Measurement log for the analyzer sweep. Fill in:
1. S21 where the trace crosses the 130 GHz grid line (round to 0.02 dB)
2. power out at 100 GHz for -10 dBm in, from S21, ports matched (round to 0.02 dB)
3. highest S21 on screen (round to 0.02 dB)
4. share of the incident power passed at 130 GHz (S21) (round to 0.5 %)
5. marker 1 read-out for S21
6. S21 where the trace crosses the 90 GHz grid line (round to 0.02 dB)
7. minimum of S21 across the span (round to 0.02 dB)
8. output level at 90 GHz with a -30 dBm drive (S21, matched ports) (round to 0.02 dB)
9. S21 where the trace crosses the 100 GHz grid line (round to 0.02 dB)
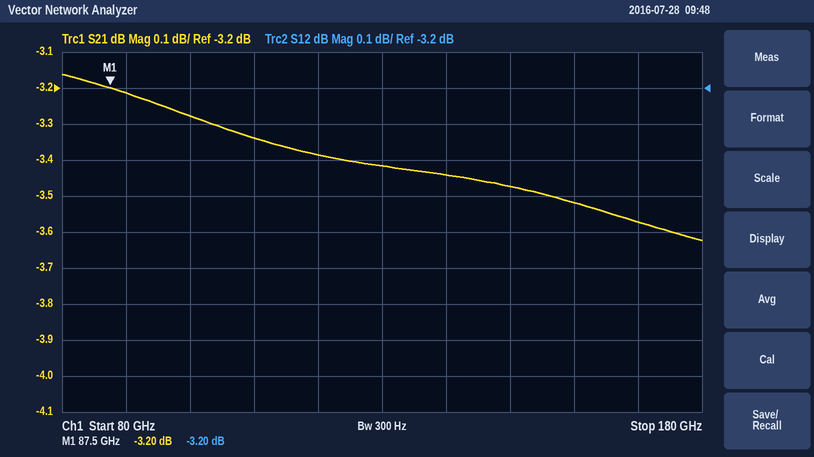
-3.42 dB
-13.28 dBm
-3.16 dB
45.5 %
-3.20 dB
-3.22 dB
-3.62 dB
-33.22 dBm
-3.28 dB
